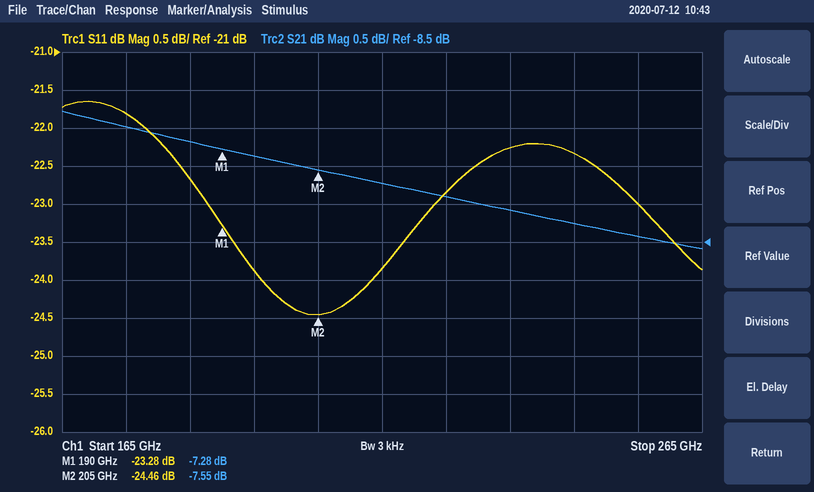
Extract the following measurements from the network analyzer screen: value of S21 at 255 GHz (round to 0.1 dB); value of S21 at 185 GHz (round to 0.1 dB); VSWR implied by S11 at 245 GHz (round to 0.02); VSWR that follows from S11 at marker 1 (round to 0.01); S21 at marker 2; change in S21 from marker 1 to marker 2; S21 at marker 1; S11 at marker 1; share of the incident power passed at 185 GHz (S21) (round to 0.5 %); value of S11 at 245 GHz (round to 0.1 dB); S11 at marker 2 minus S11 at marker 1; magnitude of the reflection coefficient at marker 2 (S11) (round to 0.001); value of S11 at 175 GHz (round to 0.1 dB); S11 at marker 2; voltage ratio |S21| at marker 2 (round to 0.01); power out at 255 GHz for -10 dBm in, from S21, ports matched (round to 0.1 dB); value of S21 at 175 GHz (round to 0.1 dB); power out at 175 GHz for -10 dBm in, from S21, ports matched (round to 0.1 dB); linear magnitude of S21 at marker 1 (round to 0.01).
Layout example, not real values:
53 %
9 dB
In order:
-8.4 dB
-7.2 dB
1.16
1.15
-7.55 dB
-0.27 dB
-7.28 dB
-23.28 dB
19.0 %
-22.3 dB
-1.18 dB
0.060
-21.8 dB
-24.46 dB
0.42
-18.4 dBm
-7.0 dB
-17.0 dBm
0.43
